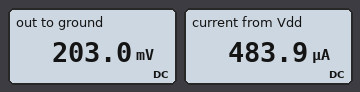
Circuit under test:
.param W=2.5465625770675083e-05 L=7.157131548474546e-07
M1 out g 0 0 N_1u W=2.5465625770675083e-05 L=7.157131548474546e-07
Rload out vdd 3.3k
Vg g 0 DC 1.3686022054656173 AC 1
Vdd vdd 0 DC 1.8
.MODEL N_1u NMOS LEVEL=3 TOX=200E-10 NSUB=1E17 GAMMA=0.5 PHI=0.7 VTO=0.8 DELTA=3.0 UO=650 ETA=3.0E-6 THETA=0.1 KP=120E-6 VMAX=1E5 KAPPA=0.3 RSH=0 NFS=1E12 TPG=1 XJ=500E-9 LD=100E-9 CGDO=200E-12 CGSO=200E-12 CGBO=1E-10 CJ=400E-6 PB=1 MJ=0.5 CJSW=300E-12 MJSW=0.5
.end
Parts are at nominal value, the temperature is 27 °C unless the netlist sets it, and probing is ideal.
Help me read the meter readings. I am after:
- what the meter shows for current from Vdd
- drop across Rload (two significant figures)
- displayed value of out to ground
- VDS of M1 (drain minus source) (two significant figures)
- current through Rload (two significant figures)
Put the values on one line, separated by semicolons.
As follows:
483.9 µA; 1.6 V; 203.0 mV; 200 mV; 480 µA
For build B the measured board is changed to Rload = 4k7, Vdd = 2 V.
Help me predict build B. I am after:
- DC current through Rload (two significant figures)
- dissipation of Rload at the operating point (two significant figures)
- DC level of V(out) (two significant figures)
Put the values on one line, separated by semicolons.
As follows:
390 µA; 730 µW; 150 mV
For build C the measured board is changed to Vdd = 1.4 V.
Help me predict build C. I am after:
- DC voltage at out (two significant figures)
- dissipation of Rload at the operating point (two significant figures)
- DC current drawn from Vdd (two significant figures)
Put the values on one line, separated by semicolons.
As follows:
140 mV; 480 µW; 380 µA
